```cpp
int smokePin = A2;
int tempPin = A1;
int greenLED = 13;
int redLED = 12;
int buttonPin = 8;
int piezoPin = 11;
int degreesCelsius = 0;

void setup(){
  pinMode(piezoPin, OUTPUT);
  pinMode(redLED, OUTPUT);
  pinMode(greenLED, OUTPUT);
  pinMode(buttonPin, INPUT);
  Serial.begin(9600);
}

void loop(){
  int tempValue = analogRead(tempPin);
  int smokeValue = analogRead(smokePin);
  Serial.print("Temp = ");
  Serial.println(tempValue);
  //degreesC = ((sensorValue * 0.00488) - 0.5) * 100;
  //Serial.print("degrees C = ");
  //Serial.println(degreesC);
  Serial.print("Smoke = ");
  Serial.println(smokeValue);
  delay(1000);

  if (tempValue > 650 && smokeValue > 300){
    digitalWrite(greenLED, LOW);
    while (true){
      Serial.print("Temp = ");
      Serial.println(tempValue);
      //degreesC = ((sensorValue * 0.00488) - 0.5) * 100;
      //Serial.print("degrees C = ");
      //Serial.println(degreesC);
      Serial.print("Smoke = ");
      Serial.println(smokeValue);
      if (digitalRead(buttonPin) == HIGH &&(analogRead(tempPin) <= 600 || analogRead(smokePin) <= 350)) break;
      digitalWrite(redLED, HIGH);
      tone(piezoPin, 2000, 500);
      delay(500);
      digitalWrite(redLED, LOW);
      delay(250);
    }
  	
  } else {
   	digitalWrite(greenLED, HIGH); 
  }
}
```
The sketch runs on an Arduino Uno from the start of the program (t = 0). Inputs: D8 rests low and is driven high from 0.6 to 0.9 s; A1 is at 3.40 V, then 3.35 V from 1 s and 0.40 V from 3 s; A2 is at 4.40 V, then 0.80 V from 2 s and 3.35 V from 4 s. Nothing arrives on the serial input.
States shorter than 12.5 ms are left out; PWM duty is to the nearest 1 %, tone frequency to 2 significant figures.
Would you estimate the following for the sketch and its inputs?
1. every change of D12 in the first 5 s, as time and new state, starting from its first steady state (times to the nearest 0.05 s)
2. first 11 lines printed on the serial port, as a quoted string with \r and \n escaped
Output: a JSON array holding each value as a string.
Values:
["0 s low; 1 s high; 1.5 s low; 1.75 s high; 2.25 s low; 2.5 s high; 3 s low; 3.25 s high; 3.75 s low; 4 s high; 4.5 s low; 4.75 s high", "\"Temp = 696\\r\\nSmoke = 901\\r\\nTemp = 696\\r\\nSmoke = 901\\r\\nTemp = 696\\r\\nSmoke = 901\\r\\nTemp = 696\\r\\nSmoke = 901\\r\\nTemp = 696\\r\\nSmoke = 901\\r\\nTemp = 696\\r\\n\""]
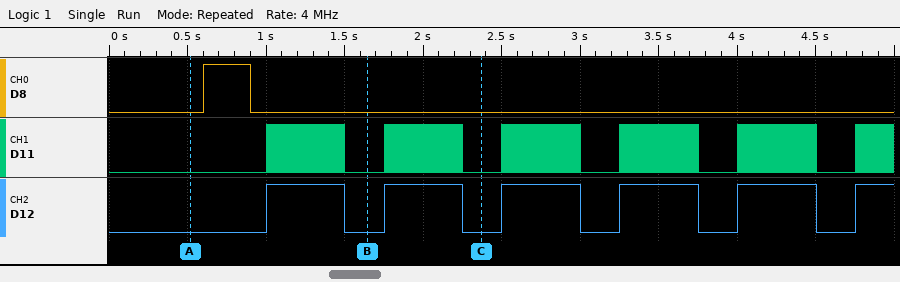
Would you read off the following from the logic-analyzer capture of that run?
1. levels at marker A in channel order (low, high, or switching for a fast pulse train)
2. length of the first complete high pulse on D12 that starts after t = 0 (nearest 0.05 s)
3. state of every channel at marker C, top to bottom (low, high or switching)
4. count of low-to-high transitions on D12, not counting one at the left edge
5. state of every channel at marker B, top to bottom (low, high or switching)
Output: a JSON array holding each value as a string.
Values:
["D8 low, D11 low, D12 low", "0.50 s", "D8 low, D11 low, D12 low", "6", "D8 low, D11 low, D12 low"]
